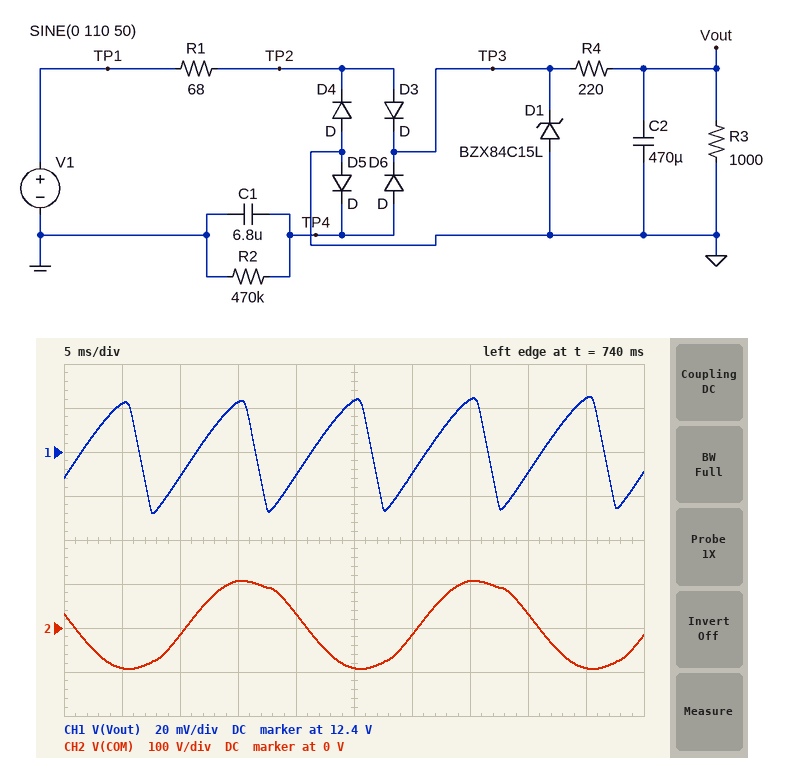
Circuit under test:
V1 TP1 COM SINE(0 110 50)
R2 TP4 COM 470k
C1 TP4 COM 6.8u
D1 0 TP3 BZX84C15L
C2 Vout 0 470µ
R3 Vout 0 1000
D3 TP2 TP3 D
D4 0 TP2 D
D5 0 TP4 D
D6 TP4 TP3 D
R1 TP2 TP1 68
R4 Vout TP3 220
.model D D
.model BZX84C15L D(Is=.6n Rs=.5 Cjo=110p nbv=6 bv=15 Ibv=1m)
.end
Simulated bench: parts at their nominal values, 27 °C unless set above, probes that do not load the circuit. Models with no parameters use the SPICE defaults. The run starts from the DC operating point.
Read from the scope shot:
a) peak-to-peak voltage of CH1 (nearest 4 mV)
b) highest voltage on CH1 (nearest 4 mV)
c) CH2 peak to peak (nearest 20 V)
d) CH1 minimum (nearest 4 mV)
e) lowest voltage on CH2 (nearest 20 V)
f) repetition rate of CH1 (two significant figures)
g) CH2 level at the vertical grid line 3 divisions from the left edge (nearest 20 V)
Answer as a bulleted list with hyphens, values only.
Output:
- 52 mV
- 12.424 V
- 200 V
- 12.372 V
- -100 V
- 100 Hz
- 100 V
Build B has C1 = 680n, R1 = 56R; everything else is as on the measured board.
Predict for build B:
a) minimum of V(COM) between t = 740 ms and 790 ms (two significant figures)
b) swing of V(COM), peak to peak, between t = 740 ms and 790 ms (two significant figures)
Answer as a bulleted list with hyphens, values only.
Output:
- -98 V
- 210 V
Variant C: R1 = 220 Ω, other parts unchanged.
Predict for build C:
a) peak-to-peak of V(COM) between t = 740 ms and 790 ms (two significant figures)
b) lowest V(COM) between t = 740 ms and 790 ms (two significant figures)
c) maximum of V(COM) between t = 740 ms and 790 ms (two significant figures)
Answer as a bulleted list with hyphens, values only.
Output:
- 180 V
- -83 V
- 98 V
